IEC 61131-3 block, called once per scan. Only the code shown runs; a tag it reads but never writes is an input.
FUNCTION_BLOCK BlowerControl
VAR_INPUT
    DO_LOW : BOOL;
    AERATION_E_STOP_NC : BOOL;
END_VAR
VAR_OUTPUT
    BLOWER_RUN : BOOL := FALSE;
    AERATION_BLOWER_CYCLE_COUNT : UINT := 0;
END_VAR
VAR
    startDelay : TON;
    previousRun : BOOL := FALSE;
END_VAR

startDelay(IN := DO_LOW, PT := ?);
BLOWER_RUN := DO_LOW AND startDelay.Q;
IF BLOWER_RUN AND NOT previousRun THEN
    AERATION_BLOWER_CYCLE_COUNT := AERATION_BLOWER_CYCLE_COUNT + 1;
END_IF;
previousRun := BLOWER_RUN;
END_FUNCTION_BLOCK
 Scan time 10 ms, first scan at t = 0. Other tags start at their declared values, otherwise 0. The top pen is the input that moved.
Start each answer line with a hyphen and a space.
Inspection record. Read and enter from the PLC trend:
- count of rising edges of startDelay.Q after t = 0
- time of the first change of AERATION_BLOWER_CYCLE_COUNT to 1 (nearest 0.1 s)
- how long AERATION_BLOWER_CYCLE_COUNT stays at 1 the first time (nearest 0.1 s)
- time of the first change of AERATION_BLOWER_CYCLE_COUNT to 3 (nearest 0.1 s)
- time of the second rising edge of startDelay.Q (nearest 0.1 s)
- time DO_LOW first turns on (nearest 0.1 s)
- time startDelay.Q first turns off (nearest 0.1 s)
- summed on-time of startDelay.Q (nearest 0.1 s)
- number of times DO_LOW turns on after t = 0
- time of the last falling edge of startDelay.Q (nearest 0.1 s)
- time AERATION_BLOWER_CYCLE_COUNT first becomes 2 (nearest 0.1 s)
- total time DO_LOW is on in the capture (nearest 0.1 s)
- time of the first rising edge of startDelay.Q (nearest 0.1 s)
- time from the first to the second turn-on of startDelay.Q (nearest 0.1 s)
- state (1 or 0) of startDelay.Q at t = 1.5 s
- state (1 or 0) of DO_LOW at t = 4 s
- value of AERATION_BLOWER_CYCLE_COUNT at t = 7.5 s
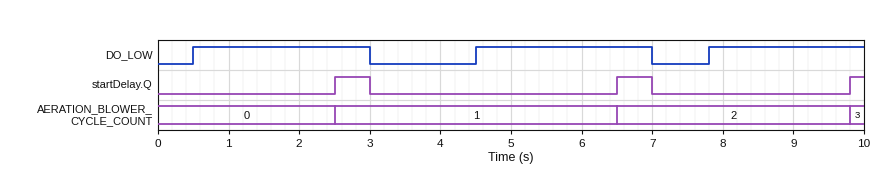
- 3
- 2.5 s
- 4.0 s
- 9.8 s
- 6.5 s
- 0.5 s
- 3.0 s
- 1.2 s
- 3
- 7.0 s
- 6.5 s
- 7.2 s
- 2.5 s
- 4.0 s
- 0
- 0
- 2
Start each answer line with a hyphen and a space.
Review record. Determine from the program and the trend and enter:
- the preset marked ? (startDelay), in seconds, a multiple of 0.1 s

- 2.0 s
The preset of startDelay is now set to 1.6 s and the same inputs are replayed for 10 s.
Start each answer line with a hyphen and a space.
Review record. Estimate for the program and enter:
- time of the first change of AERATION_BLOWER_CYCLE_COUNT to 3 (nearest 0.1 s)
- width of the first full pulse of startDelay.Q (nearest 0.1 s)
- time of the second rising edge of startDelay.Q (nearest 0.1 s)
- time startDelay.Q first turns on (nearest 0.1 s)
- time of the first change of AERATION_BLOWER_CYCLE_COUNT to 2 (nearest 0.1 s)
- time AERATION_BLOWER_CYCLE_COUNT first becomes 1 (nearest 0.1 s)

- 9.4 s
- 0.9 s
- 6.1 s
- 2.1 s
- 6.1 s
- 2.1 s
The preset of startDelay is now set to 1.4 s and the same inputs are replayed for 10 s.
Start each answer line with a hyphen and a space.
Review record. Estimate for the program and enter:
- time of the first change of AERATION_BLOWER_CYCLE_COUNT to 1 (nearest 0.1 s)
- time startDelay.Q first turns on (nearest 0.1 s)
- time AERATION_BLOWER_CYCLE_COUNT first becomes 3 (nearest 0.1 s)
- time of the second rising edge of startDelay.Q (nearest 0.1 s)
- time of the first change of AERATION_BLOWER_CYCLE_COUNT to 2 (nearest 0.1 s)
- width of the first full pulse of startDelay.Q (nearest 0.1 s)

- 1.9 s
- 1.9 s
- 9.2 s
- 5.9 s
- 5.9 s
- 1.1 s
